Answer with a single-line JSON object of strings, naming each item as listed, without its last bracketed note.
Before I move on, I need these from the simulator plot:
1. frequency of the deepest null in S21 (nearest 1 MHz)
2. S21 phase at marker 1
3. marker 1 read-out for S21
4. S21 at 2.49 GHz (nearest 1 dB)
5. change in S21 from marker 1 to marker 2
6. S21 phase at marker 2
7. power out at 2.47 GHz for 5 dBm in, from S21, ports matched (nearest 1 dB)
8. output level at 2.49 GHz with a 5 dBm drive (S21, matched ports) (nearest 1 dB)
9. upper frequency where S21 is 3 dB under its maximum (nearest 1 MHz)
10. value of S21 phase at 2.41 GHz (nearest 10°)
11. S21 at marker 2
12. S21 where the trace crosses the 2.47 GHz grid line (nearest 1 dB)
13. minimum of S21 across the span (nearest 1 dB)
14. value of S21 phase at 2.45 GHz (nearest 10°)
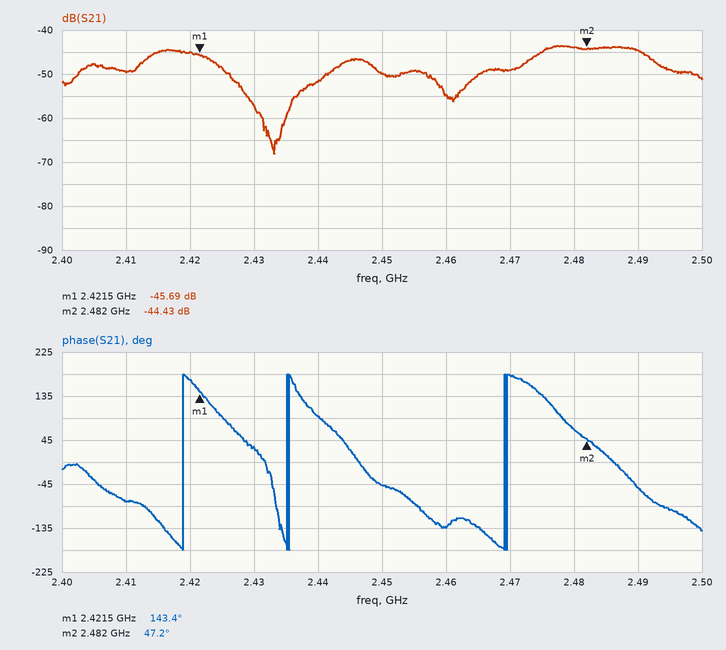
{"frequency of the deepest null in S21": "2.433 GHz", "S21 phase at marker 1": "143.4°", "marker 1 read-out for S21": "-45.69 dB", "S21 at 2.49 GHz": "-45 dB", "change in S21 from marker 1 to marker 2": "1.26 dB", "S21 phase at marker 2": "47.2°", "power out at 2.47 GHz for 5 dBm in, from S21, ports matched": "-44 dBm", "output level at 2.49 GHz with a 5 dBm drive (S21, matched ports)": "-40 dBm", "upper frequency where S21 is 3 dB under its maximum": "2.492 GHz", "value of S21 phase at 2.41 GHz": "-80°", "S21 at marker 2": "-44.43 dB", "S21 where the trace crosses the 2.47 GHz grid line": "-49 dB", "minimum of S21 across the span": "-68 dB", "value of S21 phase at 2.45 GHz": "-50°"}
